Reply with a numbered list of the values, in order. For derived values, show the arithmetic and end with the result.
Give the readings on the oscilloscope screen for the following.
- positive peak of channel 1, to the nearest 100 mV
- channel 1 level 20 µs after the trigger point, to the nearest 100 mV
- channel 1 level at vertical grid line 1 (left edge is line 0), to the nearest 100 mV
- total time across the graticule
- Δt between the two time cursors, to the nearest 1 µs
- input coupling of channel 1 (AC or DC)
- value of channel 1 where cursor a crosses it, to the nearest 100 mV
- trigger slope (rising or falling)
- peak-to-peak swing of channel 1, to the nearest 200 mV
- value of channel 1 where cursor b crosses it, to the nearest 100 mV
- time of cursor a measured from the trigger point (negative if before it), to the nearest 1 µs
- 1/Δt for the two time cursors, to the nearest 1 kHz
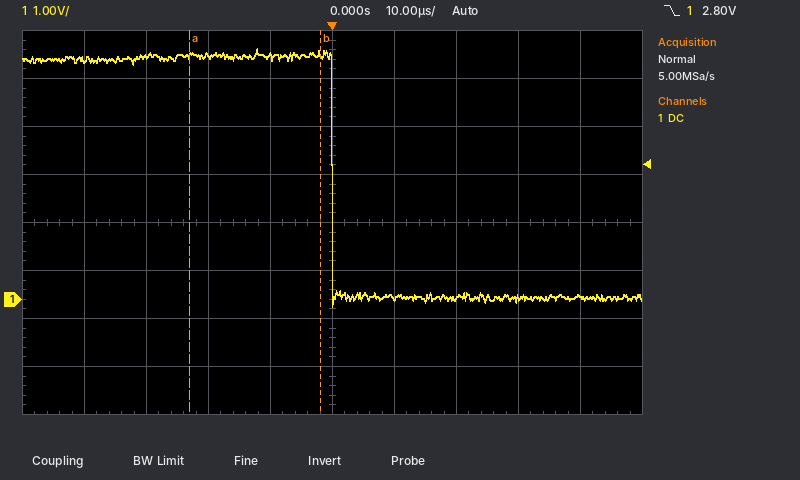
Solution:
1. 5.2 V
2. 0.0 V
3. 5.0 V
4. 100 µs
5. 21 µs
6. DC
7. 5.1 V
8. falling
9. 5.4 V
10. 5.1 V
11. -23 µs
12. 1 / 21 µs ≈ 48 kHz
